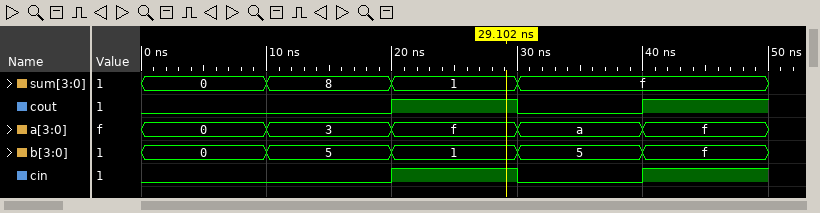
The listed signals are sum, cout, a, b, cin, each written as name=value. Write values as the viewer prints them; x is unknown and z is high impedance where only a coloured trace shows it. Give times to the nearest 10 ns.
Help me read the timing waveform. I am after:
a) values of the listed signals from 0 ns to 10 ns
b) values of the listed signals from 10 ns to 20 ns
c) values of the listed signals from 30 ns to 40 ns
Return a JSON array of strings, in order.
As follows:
["sum=0, cout=0, a=0, b=0, cin=0", "sum=8, cout=0, a=3, b=5, cin=0", "sum=f, cout=0, a=a, b=5, cin=0"]
